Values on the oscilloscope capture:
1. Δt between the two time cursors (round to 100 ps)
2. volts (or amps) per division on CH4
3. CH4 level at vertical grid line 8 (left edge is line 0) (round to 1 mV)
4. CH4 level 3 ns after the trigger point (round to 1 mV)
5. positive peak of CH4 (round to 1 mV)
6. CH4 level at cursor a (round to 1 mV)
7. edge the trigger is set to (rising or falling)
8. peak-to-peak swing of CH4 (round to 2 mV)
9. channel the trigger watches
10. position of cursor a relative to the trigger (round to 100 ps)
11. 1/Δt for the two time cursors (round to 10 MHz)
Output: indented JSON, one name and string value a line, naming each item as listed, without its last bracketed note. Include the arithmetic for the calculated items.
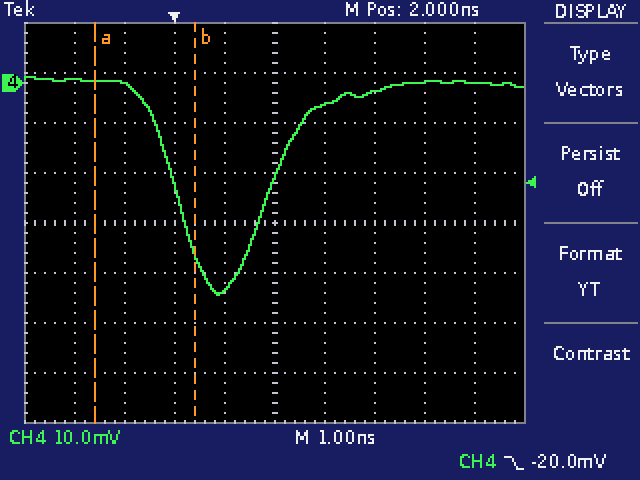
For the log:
{
  "Δt between the two time cursors": "2.0 ns",
  "volts (or amps) per division on CH4": "10 mV",
  "CH4 level at vertical grid line 8 (left edge is line 0)": "0 mV",
  "CH4 level 3 ns after the trigger point": "-4 mV",
  "positive peak of CH4": "1 mV",
  "CH4 level at cursor a": "0 mV",
  "edge the trigger is set to": "falling",
  "peak-to-peak swing of CH4": "44 mV",
  "channel the trigger watches": "CH4",
  "position of cursor a relative to the trigger": "-1.6 ns",
  "1/Δt for the two time cursors": "1 / 2.0 ns ≈ 500 MHz"
}
